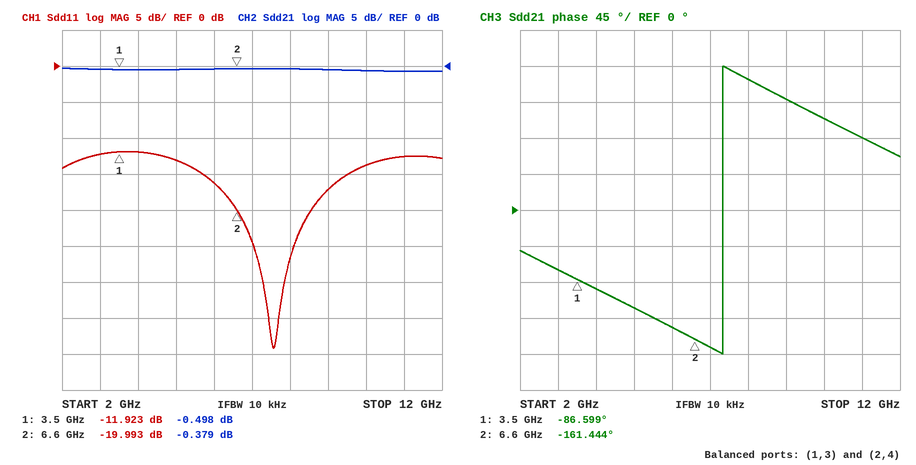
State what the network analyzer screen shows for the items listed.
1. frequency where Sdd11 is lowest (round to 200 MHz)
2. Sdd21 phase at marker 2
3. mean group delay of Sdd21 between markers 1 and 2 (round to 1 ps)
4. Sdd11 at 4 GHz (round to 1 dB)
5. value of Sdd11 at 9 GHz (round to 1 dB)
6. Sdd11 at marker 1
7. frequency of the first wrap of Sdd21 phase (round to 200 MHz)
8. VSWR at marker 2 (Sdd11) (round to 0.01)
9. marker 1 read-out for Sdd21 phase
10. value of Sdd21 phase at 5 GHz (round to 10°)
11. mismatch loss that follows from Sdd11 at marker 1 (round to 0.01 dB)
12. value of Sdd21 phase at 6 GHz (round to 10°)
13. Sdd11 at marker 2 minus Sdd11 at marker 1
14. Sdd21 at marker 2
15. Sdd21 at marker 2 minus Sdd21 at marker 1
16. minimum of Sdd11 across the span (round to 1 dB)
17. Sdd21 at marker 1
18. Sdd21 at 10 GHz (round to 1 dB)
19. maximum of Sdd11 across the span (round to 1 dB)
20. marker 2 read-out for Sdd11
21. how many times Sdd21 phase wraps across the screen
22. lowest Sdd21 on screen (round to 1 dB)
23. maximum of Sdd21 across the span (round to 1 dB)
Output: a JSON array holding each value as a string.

["7.6 GHz", "-161.444°", "67 ps", "-12 dB", "-17 dB", "-11.923 dB", "7.4 GHz", "1.22", "-86.599°", "-120°", "0.29 dB", "-150°", "-8.070 dB", "-0.379 dB", "0.119 dB", "-39 dB", "-0.498 dB", "-1 dB", "-12 dB", "-19.993 dB", "1", "-1 dB", "0 dB"]
